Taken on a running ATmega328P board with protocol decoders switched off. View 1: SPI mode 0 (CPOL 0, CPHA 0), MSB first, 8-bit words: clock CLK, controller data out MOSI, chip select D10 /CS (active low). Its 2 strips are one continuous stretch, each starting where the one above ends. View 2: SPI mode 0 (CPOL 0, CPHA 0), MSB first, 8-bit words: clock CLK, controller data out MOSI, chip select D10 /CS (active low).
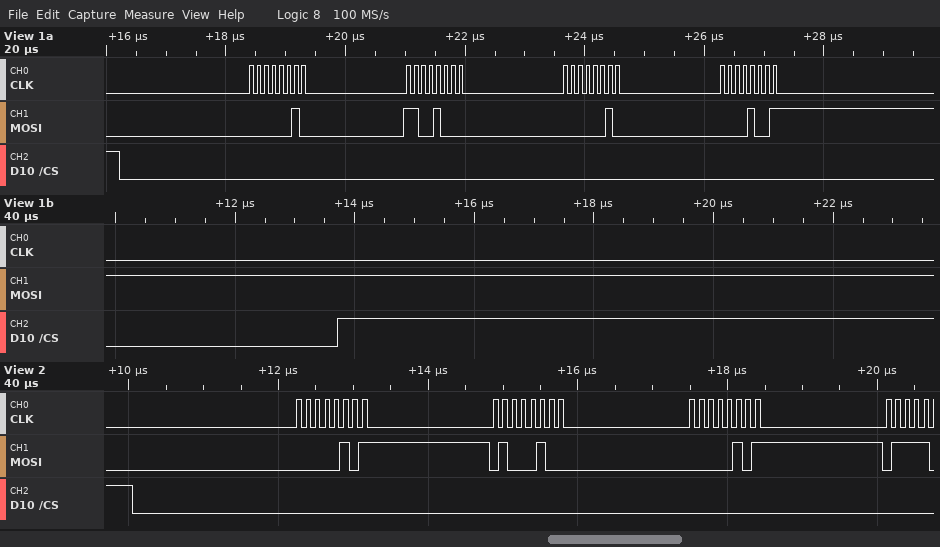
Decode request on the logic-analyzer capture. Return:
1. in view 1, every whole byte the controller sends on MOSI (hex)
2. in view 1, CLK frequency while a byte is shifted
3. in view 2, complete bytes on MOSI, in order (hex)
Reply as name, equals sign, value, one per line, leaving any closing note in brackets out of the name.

in view 1, every whole byte the controller sends on MOSI = 02 C8 02 09
in view 1, CLK frequency while a byte is shifted = 8 MHz
in view 2, complete bytes on MOSI, in order = 0x05 0x44 0x05
